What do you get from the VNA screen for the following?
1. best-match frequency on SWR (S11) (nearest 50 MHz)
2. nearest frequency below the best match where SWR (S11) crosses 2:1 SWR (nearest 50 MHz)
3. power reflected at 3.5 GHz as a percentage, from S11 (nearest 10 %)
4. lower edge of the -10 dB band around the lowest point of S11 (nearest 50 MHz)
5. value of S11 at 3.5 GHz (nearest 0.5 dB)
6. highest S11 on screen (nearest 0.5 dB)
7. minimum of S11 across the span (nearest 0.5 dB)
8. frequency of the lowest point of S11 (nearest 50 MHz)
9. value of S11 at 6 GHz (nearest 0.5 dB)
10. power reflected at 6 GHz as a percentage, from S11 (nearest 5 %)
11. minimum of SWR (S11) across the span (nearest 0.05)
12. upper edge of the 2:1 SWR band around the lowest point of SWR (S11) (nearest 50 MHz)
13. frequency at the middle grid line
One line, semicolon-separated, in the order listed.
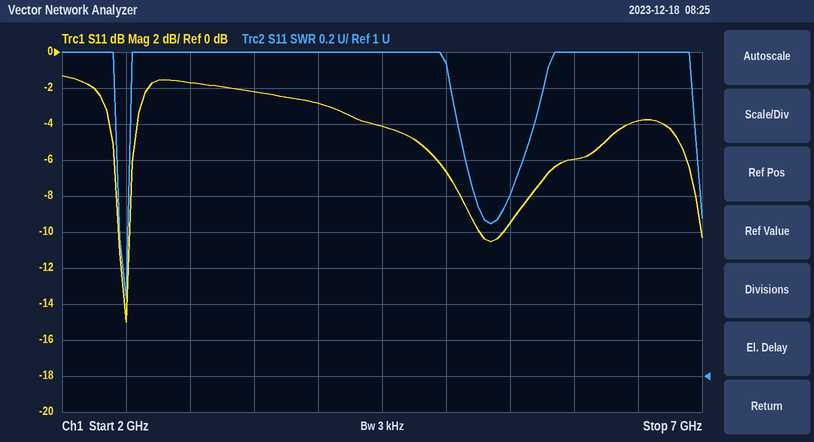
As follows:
2.50 GHz; 2.45 GHz; 60 %; 2.45 GHz; -2.0 dB; -1.5 dB; -15.0 dB; 2.50 GHz; -6.0 dB; 25 %; 1.45; 2.50 GHz; 4.5 GHz
